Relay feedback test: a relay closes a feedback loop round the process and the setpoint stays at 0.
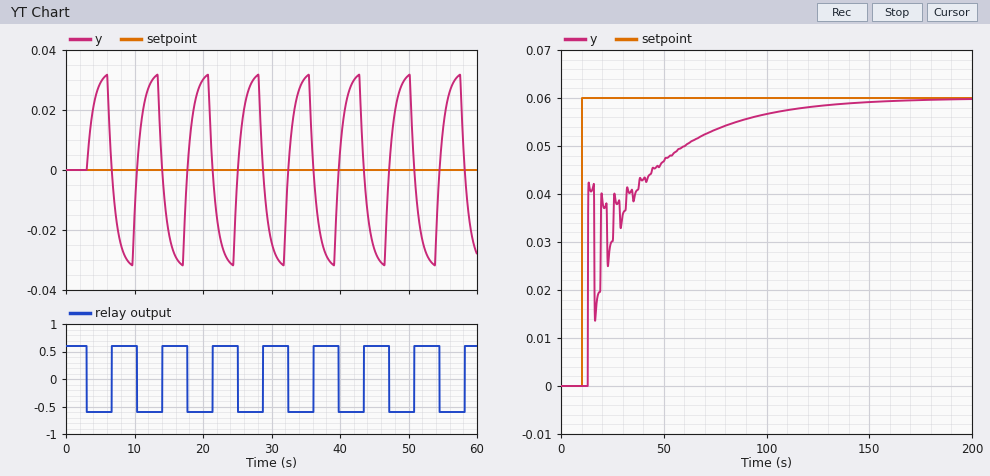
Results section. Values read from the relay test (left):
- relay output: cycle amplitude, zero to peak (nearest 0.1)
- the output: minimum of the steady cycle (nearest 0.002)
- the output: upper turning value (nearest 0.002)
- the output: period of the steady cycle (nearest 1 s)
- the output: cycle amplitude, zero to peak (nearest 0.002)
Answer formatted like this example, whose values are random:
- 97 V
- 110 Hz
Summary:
- 0.6
- -0.032
- 0.032
- 7 s
- 0.032
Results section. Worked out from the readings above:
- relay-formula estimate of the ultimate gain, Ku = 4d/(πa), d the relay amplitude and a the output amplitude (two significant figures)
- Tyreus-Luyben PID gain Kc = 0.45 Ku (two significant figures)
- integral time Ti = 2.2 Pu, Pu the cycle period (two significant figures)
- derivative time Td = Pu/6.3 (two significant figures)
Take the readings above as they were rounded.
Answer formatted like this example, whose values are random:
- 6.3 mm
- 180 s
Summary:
- 24
- 11
- 15 s
- 1.1 s
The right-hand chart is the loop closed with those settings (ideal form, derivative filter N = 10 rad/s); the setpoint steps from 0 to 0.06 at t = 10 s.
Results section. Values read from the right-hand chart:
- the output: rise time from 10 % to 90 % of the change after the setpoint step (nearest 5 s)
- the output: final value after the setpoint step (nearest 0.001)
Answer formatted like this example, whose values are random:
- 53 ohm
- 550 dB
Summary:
- 65 s
- 0.060
